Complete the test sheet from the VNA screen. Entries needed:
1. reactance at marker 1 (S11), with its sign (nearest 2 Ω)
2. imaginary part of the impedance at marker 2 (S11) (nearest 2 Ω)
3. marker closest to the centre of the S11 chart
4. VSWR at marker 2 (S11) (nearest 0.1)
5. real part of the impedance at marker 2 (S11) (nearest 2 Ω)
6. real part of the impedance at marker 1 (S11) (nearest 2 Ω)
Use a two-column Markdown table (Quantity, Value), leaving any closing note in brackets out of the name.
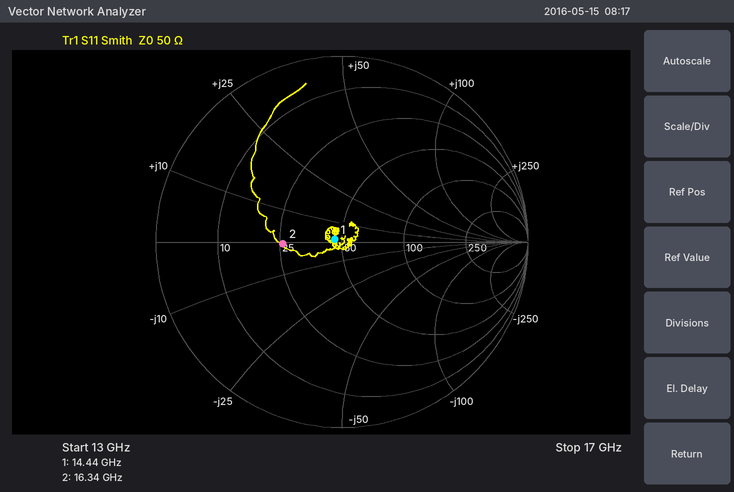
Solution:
| Quantity | Value |
|---|---|
| reactance at marker 1 (S11), with its sign | +2 Ω |
| imaginary part of the impedance at marker 2 (S11) | 0 Ω |
| marker closest to the centre of the S11 chart | marker 1 |
| VSWR at marker 2 (S11) | 1.9 |
| real part of the impedance at marker 2 (S11) | 26 Ω |
| real part of the impedance at marker 1 (S11) | 46 Ω |
